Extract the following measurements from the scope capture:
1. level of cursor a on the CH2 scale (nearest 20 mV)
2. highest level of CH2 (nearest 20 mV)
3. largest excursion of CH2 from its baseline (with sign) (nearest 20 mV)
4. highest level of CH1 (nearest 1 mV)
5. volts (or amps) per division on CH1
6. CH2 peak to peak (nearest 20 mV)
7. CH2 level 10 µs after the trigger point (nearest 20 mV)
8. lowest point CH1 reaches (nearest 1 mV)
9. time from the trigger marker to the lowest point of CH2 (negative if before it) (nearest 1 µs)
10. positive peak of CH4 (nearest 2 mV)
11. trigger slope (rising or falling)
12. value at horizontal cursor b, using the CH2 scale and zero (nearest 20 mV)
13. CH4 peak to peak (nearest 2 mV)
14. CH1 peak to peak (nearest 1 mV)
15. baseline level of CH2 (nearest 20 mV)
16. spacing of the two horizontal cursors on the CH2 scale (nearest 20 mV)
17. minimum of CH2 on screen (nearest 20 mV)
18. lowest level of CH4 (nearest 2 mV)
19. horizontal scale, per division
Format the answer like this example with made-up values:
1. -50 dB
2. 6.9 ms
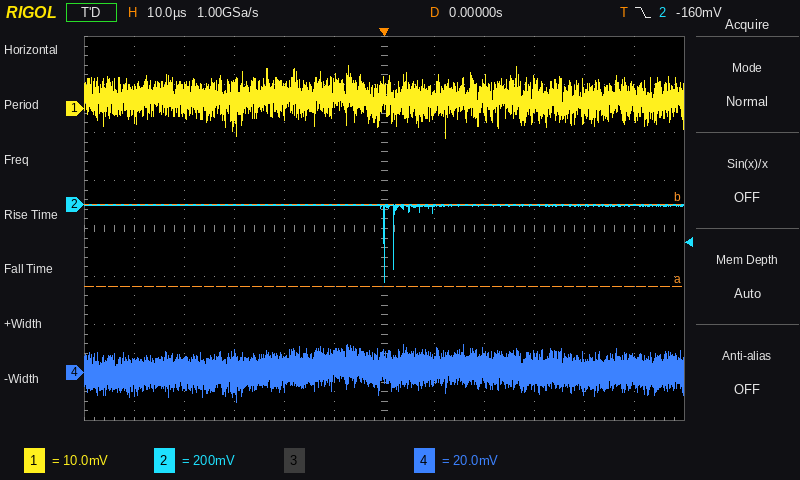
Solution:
1. -340 mV
2. 0 mV
3. -320 mV
4. 9 mV
5. 10 mV
6. 320 mV
7. -20 mV
8. -6 mV
9. 0 µs
10. 12 mV
11. falling
12. 0 mV
13. 24 mV
14. 15 mV
15. 0 mV
16. 340 mV
17. -320 mV
18. -12 mV
19. 10 µs
